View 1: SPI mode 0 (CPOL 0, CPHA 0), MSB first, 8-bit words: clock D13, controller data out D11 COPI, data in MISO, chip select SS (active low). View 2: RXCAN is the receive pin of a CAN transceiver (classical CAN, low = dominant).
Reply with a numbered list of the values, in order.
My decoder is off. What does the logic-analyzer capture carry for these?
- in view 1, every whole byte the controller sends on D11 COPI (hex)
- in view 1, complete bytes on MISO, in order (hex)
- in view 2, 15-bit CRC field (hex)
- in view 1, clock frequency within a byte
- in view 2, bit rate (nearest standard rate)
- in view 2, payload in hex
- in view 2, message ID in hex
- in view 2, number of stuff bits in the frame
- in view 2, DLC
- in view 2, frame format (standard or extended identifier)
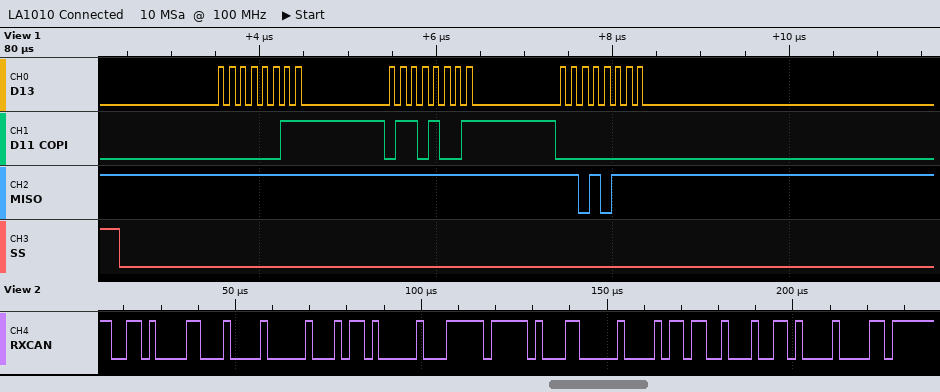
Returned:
1. 03 69 00
2. FF FF D7
3. 0x3421
4. 8 MHz
5. 500 kbit/s
6. 40 2D 00 FF E3 00 5B 22
7. 0x343
8. 5
9. 8
10. standard
